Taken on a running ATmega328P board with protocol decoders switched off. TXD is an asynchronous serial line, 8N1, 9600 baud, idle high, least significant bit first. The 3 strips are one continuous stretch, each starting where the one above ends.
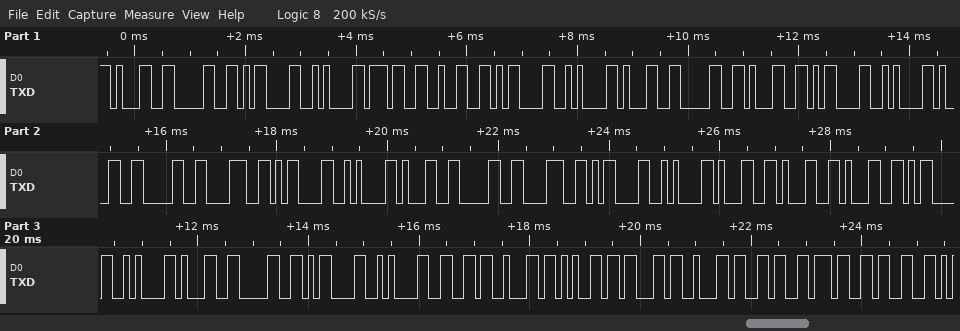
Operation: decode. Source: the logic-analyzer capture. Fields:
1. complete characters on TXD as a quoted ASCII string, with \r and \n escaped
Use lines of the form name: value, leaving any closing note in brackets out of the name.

complete characters on TXD as a quoted ASCII string, with \r and \n escaped: "10\r\n72\r\n101\r\n108\r\n108\r\n111\r\n10\r\nfbecb673"
